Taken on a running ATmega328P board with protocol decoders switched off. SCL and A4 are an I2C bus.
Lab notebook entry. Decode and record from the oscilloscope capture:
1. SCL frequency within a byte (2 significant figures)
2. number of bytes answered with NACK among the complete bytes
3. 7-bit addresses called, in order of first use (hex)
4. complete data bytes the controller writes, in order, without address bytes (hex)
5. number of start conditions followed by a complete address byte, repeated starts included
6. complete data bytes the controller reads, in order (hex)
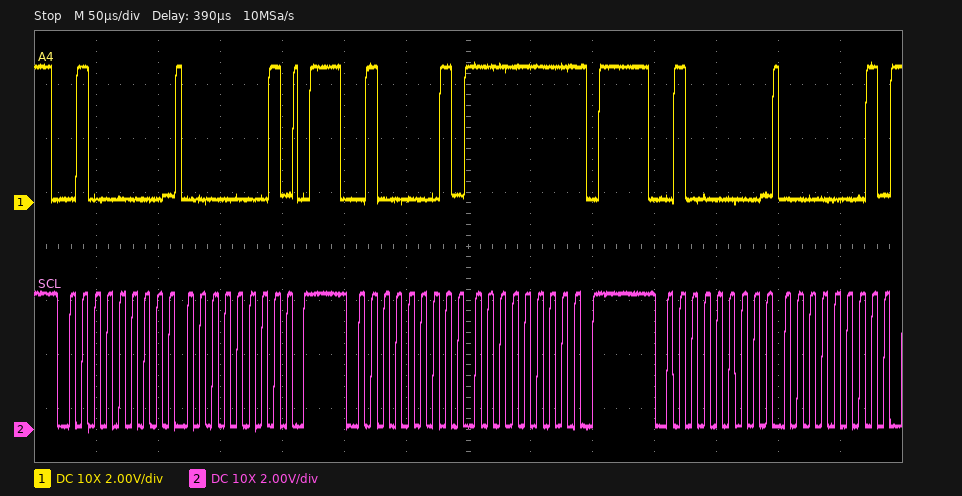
100 kHz
1
0x20
01 01
3
FF
